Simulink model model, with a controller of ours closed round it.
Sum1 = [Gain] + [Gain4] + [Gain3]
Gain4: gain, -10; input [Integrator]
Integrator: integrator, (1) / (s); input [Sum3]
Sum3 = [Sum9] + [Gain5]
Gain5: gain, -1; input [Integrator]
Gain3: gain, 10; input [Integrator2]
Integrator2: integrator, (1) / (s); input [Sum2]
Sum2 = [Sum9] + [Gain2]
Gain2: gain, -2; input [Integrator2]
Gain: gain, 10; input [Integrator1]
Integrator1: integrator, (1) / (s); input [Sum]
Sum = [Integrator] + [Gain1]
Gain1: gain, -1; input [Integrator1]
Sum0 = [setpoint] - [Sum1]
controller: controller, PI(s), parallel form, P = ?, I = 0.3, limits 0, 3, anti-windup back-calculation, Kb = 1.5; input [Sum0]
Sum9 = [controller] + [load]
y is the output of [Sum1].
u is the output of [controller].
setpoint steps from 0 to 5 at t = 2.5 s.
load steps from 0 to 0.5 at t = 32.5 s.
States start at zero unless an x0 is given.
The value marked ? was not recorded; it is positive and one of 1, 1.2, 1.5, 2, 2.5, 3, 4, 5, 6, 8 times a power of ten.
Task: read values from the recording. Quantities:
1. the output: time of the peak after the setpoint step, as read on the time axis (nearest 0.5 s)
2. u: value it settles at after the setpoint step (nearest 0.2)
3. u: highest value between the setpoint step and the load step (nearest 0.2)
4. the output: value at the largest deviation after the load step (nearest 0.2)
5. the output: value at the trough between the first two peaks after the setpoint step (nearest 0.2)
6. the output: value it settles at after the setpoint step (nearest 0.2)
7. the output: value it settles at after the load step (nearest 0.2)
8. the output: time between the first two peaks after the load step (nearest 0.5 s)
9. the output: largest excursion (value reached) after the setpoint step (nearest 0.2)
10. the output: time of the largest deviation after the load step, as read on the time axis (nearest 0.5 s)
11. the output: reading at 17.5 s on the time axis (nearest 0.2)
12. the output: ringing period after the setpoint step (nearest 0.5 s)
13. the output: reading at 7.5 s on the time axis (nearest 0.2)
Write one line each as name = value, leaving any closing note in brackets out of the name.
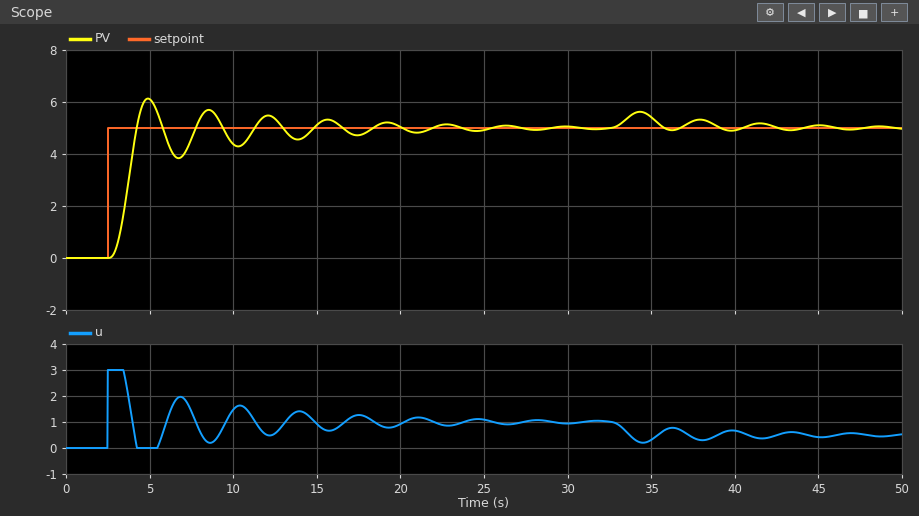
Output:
the output: time of the peak after the setpoint step, as read on the time axis = 5.0 s
u: value it settles at after the setpoint step = 1.0
u: highest value between the setpoint step and the load step = 3.0
the output: value at the largest deviation after the load step = 5.6
the output: value at the trough between the first two peaks after the setpoint step = 3.8
the output: value it settles at after the setpoint step = 5.0
the output: value it settles at after the load step = 5.0
the output: time between the first two peaks after the load step = 3.5 s
the output: largest excursion (value reached) after the setpoint step = 6.2
the output: time of the largest deviation after the load step, as read on the time axis = 34.5 s
the output: reading at 17.5 s on the time axis = 4.8
the output: ringing period after the setpoint step = 3.5 s
the output: reading at 7.5 s on the time axis = 4.6
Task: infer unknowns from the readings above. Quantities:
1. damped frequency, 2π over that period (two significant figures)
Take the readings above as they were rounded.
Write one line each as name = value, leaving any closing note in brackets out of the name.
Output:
damped frequency, 2π over that period = 1.8 rad/s
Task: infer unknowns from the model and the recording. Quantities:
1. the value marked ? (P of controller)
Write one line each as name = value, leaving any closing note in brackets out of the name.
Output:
the value marked ? = 1
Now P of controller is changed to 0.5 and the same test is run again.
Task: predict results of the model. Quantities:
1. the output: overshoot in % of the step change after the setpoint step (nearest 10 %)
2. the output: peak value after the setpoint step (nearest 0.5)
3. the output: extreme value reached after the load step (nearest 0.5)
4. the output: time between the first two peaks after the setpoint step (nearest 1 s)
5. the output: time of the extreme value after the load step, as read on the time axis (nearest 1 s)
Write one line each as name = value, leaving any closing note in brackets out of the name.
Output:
the output: overshoot in % of the step change after the setpoint step = 50 %
the output: peak value after the setpoint step = 7.5
the output: extreme value reached after the load step = 6.0
the output: time between the first two peaks after the setpoint step = 5 s
the output: time of the extreme value after the load step, as read on the time axis = 35 s
